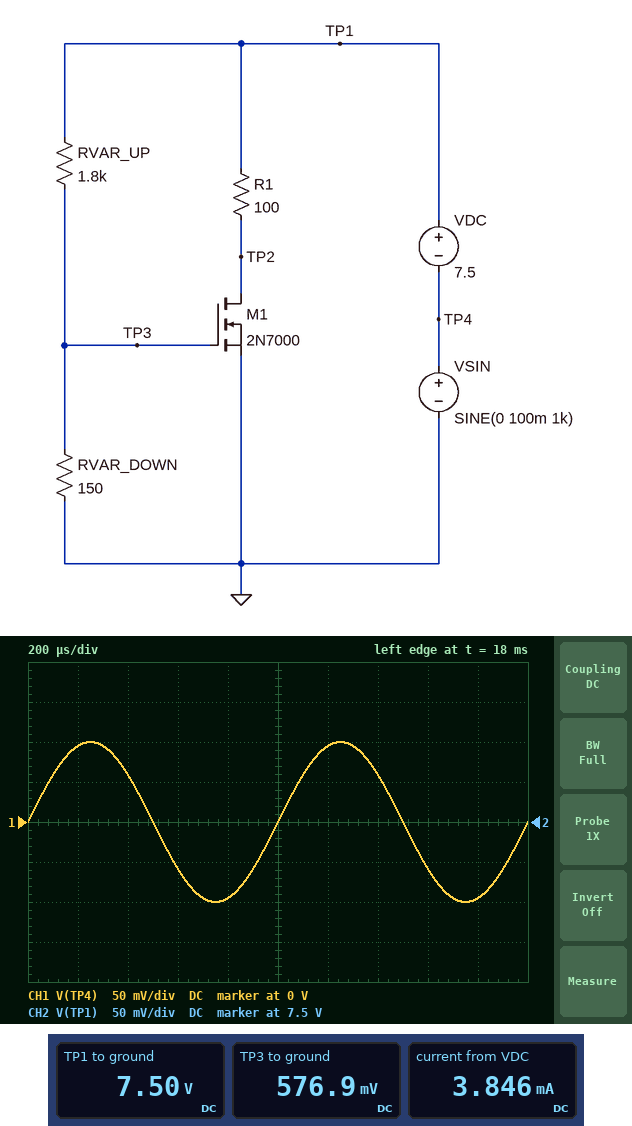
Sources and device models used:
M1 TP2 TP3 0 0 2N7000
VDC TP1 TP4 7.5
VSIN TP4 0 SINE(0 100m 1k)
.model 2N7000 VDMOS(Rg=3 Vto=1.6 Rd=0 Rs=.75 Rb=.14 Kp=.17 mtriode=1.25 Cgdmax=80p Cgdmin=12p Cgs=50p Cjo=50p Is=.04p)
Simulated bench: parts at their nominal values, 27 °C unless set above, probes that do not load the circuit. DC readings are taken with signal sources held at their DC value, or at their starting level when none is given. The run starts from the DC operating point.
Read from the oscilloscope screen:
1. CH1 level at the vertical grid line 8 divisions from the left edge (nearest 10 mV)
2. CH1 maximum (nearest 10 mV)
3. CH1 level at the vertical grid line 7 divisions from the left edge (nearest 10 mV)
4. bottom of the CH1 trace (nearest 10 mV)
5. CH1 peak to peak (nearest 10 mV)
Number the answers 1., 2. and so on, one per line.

1. -60 mV
2. 100 mV
3. 60 mV
4. -100 mV
5. 200 mV
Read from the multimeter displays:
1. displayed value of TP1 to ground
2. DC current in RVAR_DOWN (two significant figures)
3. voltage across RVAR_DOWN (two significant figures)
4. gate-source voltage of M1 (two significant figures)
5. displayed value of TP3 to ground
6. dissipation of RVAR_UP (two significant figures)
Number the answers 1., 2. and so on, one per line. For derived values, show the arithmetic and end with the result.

1. 7.50 V
2. (576.9 mV) / 150 Ω = 3.8 mA
3. 576.9 mV = 580 mV
4. 576.9 mV = 580 mV
5. 576.9 mV
6. (7.5 V - 576.9 mV)^2 / 1.8 kΩ = 27 mW
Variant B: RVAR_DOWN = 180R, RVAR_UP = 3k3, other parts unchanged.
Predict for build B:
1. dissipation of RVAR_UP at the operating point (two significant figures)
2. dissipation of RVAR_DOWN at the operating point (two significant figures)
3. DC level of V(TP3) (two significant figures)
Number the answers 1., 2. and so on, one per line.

1. 15 mW
2. 840 µW
3. 390 mV
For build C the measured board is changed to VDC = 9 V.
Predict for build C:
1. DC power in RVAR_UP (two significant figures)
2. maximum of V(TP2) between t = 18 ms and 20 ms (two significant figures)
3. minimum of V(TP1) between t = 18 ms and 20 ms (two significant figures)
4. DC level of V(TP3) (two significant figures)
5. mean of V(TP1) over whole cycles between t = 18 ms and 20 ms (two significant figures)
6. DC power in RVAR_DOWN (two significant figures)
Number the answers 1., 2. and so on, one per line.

1. 38 mW
2. 9.1 V
3. 8.9 V
4. 690 mV
5. 9.0 V
6. 3.2 mW
